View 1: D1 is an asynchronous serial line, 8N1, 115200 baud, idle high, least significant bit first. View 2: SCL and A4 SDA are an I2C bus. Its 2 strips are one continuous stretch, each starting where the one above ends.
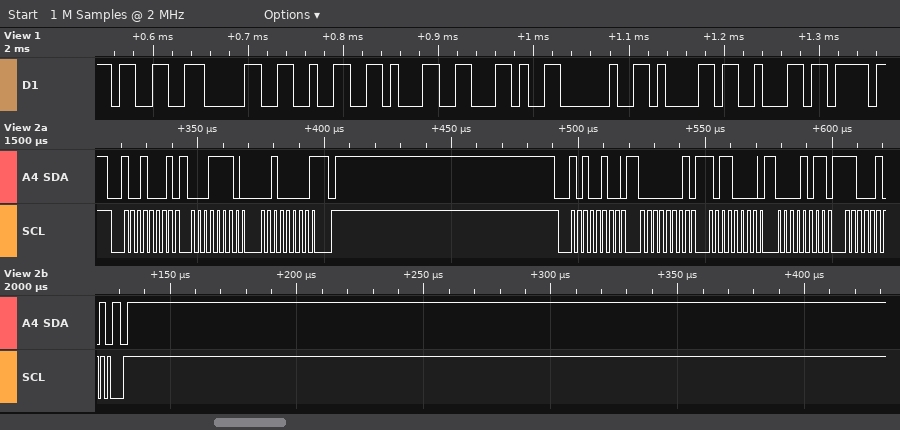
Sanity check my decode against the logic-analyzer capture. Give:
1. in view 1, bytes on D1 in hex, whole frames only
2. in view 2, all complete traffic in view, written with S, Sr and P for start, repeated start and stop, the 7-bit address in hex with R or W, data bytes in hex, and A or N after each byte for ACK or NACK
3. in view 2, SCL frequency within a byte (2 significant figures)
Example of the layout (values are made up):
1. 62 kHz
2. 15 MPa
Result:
1. 33 30 32 31 2C 20 61 62
2. S 48R A 1E A 20 N P S 52W A 01 A B0 A 0B A C5 A P
3. 400 kHz
